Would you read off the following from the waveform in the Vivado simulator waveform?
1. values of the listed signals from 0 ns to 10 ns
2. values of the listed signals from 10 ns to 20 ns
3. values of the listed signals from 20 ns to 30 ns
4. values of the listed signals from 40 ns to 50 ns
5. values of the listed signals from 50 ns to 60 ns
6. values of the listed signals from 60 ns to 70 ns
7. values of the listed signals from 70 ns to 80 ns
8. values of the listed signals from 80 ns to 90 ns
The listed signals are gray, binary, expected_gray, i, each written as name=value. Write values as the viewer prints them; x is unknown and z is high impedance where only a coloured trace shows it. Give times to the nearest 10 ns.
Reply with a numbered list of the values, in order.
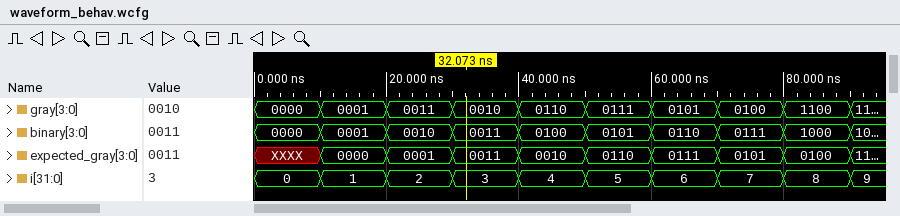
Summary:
1. gray=0000, binary=0000, expected_gray=XXXX, i=0
2. gray=0001, binary=0001, expected_gray=0000, i=1
3. gray=0011, binary=0010, expected_gray=0001, i=2
4. gray=0110, binary=0100, expected_gray=0010, i=4
5. gray=0111, binary=0101, expected_gray=0110, i=5
6. gray=0101, binary=0110, expected_gray=0111, i=6
7. gray=0100, binary=0111, expected_gray=0101, i=7
8. gray=1100, binary=1000, expected_gray=0100, i=8
